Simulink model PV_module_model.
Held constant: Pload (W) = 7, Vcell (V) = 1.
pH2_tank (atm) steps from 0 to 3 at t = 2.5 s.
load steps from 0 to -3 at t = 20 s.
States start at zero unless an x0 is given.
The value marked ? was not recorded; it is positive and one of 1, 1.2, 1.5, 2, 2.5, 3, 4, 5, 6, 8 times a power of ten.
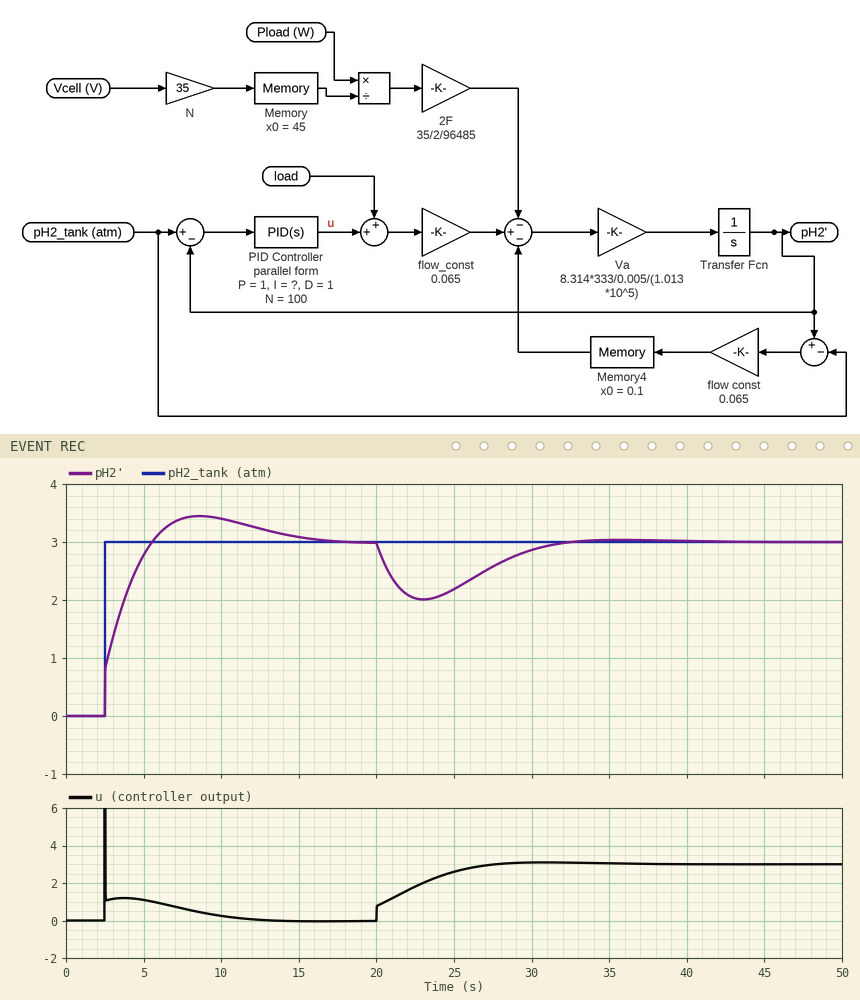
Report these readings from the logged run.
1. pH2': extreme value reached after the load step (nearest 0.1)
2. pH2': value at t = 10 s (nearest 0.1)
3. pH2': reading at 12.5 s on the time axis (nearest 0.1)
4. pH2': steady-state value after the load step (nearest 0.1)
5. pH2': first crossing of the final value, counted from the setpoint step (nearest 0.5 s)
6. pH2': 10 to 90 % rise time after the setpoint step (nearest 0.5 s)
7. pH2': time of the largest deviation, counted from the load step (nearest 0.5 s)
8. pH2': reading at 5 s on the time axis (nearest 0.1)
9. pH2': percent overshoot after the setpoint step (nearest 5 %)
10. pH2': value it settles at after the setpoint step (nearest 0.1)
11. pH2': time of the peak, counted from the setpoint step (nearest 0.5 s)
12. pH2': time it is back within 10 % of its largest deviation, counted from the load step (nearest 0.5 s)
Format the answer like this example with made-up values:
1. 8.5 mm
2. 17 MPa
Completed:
1. 2.0
2. 3.4
3. 3.2
4. 3.0
5. 3.0 s
6. 2.5 s
7. 3.0 s
8. 2.8
9. 15 %
10. 3.0
11. 6.0 s
12. 10.5 s
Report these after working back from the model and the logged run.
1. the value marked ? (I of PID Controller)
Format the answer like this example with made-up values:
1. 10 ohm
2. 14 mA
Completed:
1. 0.5
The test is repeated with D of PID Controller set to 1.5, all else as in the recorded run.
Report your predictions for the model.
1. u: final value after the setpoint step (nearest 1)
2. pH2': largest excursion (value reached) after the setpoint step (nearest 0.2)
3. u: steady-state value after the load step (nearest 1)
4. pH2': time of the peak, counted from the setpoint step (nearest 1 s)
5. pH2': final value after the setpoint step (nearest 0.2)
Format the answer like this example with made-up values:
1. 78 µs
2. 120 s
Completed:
1. 0
2. 3.4
3. 3
4. 7 s
5. 3.0
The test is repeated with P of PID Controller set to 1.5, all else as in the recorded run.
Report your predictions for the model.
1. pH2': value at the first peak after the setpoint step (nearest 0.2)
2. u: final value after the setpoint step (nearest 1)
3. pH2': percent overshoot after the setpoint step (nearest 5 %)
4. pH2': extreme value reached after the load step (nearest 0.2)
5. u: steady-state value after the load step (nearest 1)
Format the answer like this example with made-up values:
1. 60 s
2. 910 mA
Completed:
1. 3.4
2. 0
3. 10 %
4. 2.2
5. 3
